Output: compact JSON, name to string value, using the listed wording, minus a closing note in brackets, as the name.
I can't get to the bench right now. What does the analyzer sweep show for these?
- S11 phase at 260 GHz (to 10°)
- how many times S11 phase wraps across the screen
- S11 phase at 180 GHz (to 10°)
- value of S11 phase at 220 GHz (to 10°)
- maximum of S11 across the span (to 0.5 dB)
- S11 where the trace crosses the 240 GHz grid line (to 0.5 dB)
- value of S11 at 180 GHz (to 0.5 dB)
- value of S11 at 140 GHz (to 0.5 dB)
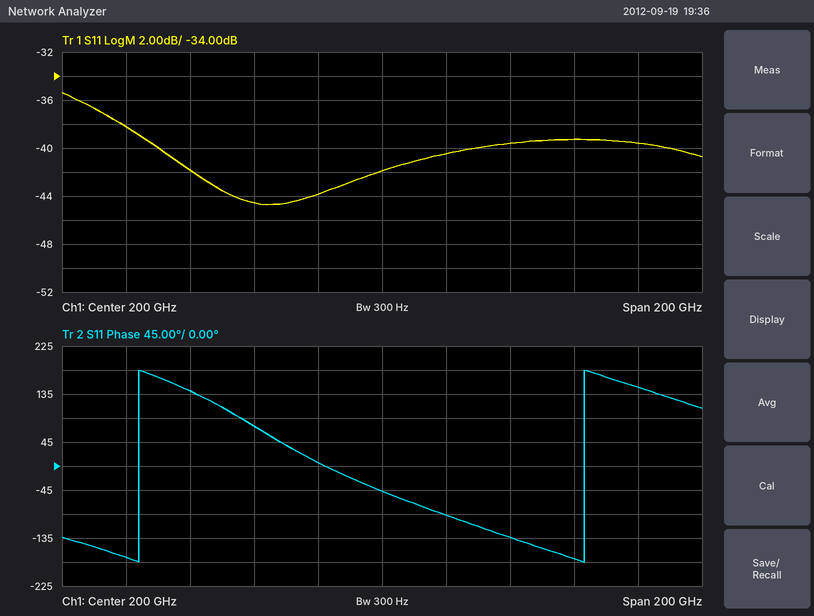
{"S11 phase at 260 GHz": "-170°", "how many times S11 phase wraps across the screen": "2", "S11 phase at 180 GHz": "10°", "value of S11 phase at 220 GHz": "-90°", "maximum of S11 across the span": "-35.5 dB", "S11 where the trace crosses the 240 GHz grid line": "-39.5 dB", "value of S11 at 180 GHz": "-44.0 dB", "value of S11 at 140 GHz": "-42.0 dB"}
